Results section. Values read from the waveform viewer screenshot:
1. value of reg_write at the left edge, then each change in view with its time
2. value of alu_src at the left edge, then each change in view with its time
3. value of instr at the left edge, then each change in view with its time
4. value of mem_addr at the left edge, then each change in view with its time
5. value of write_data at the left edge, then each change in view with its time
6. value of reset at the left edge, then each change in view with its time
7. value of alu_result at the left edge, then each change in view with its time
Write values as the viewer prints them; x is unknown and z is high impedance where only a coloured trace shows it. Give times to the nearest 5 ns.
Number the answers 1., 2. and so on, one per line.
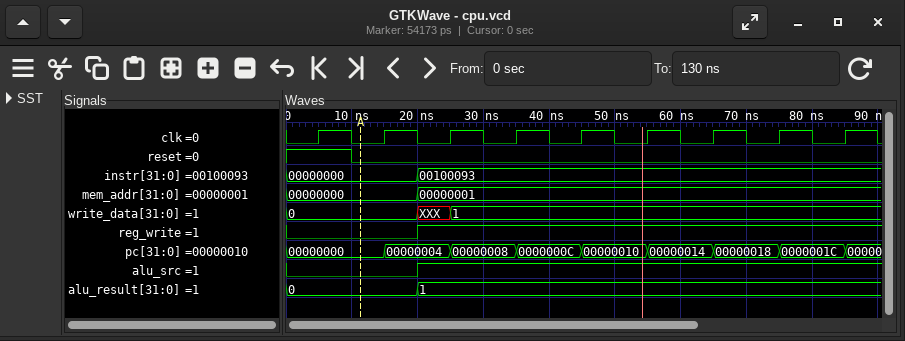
1. 0, 1 at 20 ns
2. 0, 1 at 20 ns
3. 00000000, 00100093 at 20 ns
4. 00000000, 00000001 at 20 ns
5. 0, XXX at 20 ns, 1 at 25 ns
6. 1, 0 at 10 ns
7. 0, 1 at 20 ns
